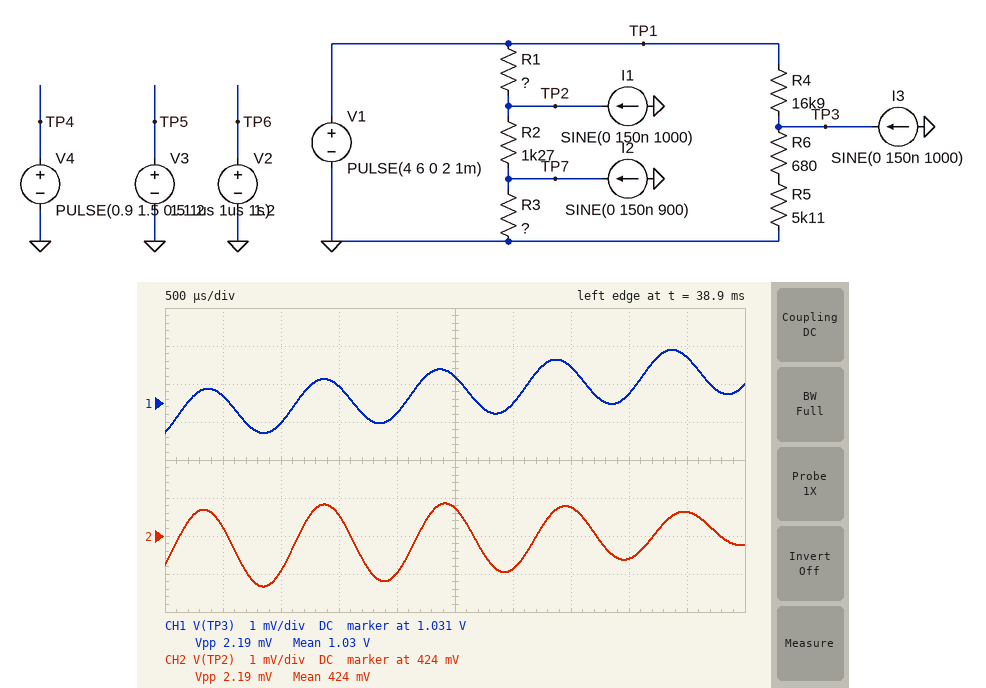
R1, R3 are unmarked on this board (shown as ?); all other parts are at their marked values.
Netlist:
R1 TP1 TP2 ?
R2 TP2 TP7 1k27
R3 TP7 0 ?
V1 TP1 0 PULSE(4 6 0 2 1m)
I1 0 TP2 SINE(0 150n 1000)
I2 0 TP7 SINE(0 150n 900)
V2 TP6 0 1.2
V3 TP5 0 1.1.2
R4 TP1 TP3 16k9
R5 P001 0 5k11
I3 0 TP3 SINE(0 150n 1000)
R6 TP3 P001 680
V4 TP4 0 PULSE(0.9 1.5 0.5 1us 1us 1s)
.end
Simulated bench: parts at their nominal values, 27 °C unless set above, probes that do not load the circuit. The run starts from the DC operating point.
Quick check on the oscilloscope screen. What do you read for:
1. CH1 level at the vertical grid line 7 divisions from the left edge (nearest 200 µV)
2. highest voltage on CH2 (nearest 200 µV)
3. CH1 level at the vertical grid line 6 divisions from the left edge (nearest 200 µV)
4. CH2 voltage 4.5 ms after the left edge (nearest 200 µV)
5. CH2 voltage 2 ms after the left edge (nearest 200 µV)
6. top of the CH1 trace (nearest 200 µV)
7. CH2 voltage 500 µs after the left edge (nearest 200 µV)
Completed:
1.0320 V
424.8 mV
1.0310 V
424.6 mV
423.0 mV
1.0324 V
424.2 mV
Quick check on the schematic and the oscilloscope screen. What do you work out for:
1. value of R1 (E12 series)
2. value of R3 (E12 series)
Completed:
39 kΩ
3.3 kΩ
